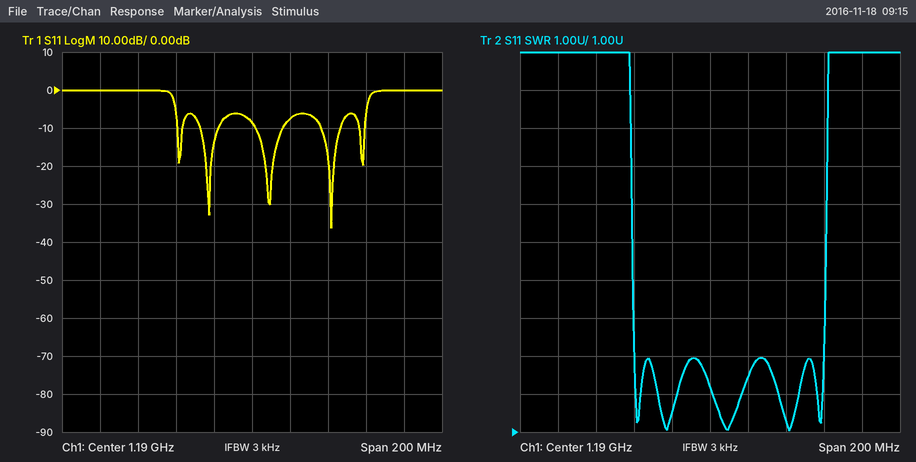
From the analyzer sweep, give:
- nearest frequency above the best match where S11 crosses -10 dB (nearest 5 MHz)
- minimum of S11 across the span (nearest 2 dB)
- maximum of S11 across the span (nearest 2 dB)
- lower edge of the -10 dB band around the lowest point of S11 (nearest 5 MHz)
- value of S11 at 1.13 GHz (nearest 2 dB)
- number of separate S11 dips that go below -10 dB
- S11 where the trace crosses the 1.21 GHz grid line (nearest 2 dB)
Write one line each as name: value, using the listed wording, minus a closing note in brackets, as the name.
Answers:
nearest frequency above the best match where S11 crosses -10 dB: 1.235 GHz
minimum of S11 across the span: -36 dB
maximum of S11 across the span: 0 dB
lower edge of the -10 dB band around the lowest point of S11: 1.225 GHz
value of S11 at 1.13 GHz: 0 dB
number of separate S11 dips that go below -10 dB: 5
S11 where the trace crosses the 1.21 GHz grid line: -8 dB
